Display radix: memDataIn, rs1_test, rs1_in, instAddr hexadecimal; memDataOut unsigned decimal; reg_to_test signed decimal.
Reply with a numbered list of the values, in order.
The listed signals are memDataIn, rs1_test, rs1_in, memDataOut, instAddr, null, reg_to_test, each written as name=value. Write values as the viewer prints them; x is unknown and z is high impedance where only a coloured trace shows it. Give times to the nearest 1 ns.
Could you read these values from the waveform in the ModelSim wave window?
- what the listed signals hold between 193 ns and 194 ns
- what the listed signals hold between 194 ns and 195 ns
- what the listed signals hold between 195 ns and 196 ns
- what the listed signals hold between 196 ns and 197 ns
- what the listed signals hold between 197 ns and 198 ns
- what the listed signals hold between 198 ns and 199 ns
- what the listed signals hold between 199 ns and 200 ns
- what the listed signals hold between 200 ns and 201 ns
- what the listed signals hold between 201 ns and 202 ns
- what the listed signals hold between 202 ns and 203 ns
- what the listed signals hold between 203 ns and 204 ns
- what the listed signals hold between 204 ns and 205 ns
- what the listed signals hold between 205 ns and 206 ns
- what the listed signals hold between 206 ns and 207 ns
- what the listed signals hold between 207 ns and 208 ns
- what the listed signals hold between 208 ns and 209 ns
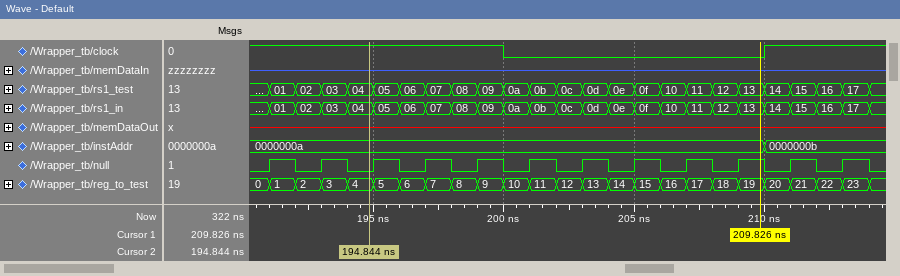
1. memDataIn=z, rs1_test=03, rs1_in=03, memDataOut=x, instAddr=0000000a, null=1, reg_to_test=3
2. memDataIn=z, rs1_test=04, rs1_in=04, memDataOut=x, instAddr=0000000a, null=0, reg_to_test=4
3. memDataIn=z, rs1_test=05, rs1_in=05, memDataOut=x, instAddr=0000000a, null=1, reg_to_test=5
4. memDataIn=z, rs1_test=06, rs1_in=06, memDataOut=x, instAddr=0000000a, null=0, reg_to_test=6
5. memDataIn=z, rs1_test=07, rs1_in=07, memDataOut=x, instAddr=0000000a, null=1, reg_to_test=7
6. memDataIn=z, rs1_test=08, rs1_in=08, memDataOut=x, instAddr=0000000a, null=0, reg_to_test=8
7. memDataIn=z, rs1_test=09, rs1_in=09, memDataOut=x, instAddr=0000000a, null=1, reg_to_test=9
8. memDataIn=z, rs1_test=0a, rs1_in=0a, memDataOut=x, instAddr=0000000a, null=0, reg_to_test=10
9. memDataIn=z, rs1_test=0b, rs1_in=0b, memDataOut=x, instAddr=0000000a, null=1, reg_to_test=11
10. memDataIn=z, rs1_test=0c, rs1_in=0c, memDataOut=x, instAddr=0000000a, null=0, reg_to_test=12
11. memDataIn=z, rs1_test=0d, rs1_in=0d, memDataOut=x, instAddr=0000000a, null=1, reg_to_test=13
12. memDataIn=z, rs1_test=0e, rs1_in=0e, memDataOut=x, instAddr=0000000a, null=0, reg_to_test=14
13. memDataIn=z, rs1_test=0f, rs1_in=0f, memDataOut=x, instAddr=0000000a, null=1, reg_to_test=15
14. memDataIn=z, rs1_test=10, rs1_in=10, memDataOut=x, instAddr=0000000a, null=0, reg_to_test=16
15. memDataIn=z, rs1_test=11, rs1_in=11, memDataOut=x, instAddr=0000000a, null=1, reg_to_test=17
16. memDataIn=z, rs1_test=12, rs1_in=12, memDataOut=x, instAddr=0000000a, null=0, reg_to_test=18
